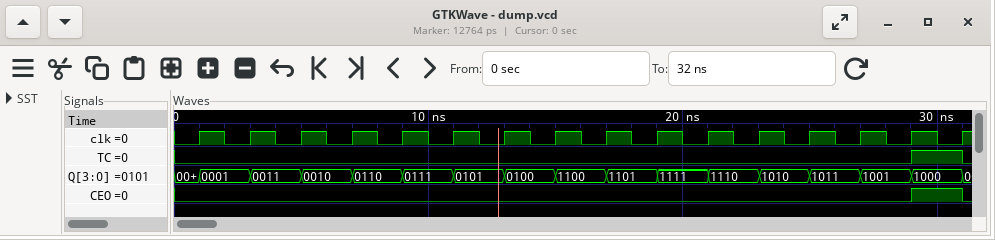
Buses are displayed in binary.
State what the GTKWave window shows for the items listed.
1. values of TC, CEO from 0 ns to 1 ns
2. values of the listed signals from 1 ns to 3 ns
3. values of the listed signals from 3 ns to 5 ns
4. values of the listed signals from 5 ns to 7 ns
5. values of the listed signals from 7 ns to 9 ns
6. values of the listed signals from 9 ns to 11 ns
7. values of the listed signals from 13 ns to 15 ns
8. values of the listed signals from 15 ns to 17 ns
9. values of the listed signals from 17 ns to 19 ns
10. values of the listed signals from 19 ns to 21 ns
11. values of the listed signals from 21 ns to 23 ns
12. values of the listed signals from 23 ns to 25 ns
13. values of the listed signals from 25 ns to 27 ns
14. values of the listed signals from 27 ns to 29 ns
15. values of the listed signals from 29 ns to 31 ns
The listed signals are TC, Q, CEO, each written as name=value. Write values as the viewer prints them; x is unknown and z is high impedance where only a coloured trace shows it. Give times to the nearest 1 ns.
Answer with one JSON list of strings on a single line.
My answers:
["TC=0, CEO=0", "TC=0, Q=0001, CEO=0", "TC=0, Q=0011, CEO=0", "TC=0, Q=0010, CEO=0", "TC=0, Q=0110, CEO=0", "TC=0, Q=0111, CEO=0", "TC=0, Q=0100, CEO=0", "TC=0, Q=1100, CEO=0", "TC=0, Q=1101, CEO=0", "TC=0, Q=1111, CEO=0", "TC=0, Q=1110, CEO=0", "TC=0, Q=1010, CEO=0", "TC=0, Q=1011, CEO=0", "TC=0, Q=1001, CEO=0", "TC=1, Q=1000, CEO=1"]
